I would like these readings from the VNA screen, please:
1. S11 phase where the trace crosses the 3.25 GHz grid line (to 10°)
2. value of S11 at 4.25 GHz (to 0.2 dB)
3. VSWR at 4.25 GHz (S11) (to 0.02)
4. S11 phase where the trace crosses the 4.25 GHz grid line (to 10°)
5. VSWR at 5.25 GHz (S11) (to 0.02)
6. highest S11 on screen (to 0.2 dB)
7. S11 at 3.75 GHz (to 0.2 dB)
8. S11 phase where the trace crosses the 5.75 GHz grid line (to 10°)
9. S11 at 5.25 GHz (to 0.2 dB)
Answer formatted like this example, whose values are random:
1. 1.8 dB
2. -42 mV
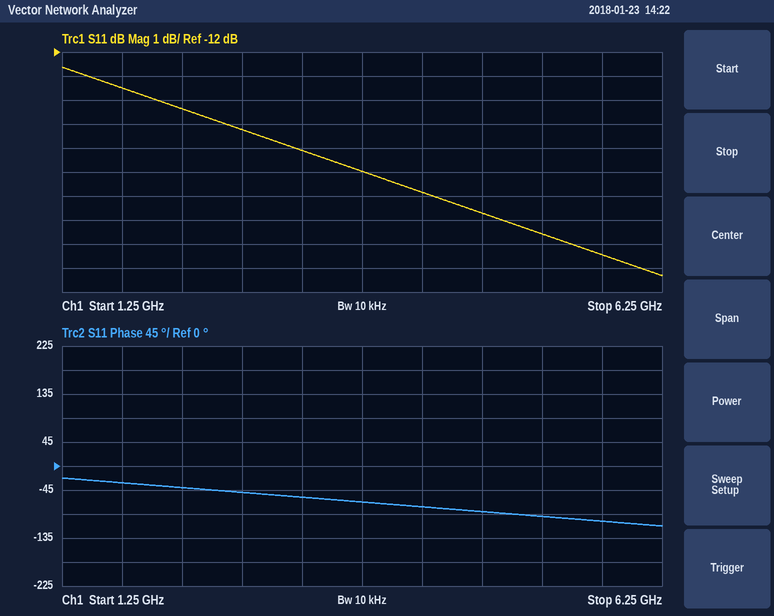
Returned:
1. -60°
2. -17.8 dB
3. 1.30
4. -80°
5. 1.24
6. -12.6 dB
7. -17.0 dB
8. -100°
9. -19.6 dB
